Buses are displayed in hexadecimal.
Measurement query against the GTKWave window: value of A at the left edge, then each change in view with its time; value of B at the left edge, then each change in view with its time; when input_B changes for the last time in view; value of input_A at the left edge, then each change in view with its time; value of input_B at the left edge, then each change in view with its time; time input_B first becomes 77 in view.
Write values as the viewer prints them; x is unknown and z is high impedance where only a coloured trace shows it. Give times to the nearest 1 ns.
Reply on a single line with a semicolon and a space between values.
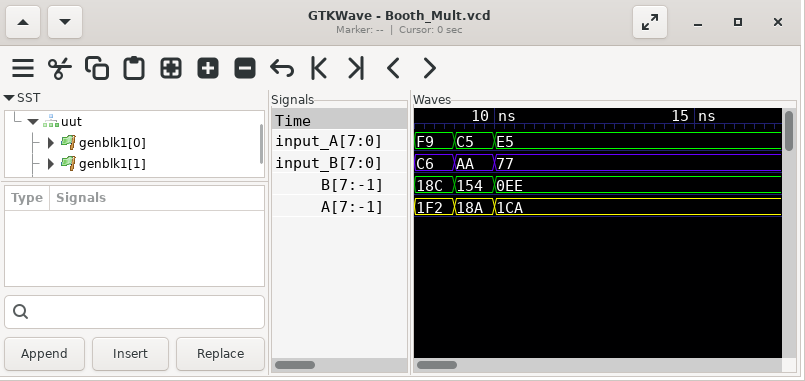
1F2, 18A at 9 ns, 1CA at 10 ns; 18C, 154 at 9 ns, 0EE at 10 ns; 10 ns; F9, C5 at 9 ns, E5 at 10 ns; C6, AA at 9 ns, 77 at 10 ns; 10 ns
